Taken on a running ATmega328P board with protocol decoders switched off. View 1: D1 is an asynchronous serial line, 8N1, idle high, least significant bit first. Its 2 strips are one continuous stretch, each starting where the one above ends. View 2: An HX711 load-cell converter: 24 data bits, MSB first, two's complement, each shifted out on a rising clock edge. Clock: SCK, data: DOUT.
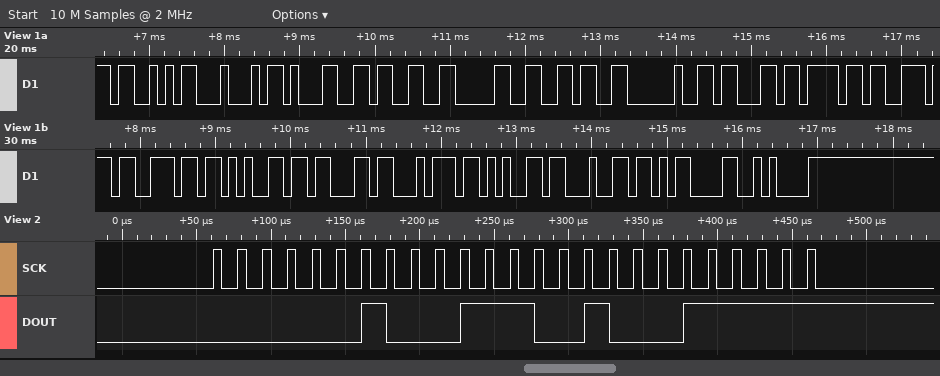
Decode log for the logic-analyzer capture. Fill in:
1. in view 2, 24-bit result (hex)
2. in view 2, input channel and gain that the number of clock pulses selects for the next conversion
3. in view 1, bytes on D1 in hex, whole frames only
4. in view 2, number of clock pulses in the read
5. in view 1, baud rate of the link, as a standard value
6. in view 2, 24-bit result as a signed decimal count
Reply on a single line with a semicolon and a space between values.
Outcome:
0x02391F; channel A, gain 128; 53 44 31 33 30 36 20 63 6F 6E 6E 65 63 74 65 64 0D 0A; 25; 9600 baud; 145695
